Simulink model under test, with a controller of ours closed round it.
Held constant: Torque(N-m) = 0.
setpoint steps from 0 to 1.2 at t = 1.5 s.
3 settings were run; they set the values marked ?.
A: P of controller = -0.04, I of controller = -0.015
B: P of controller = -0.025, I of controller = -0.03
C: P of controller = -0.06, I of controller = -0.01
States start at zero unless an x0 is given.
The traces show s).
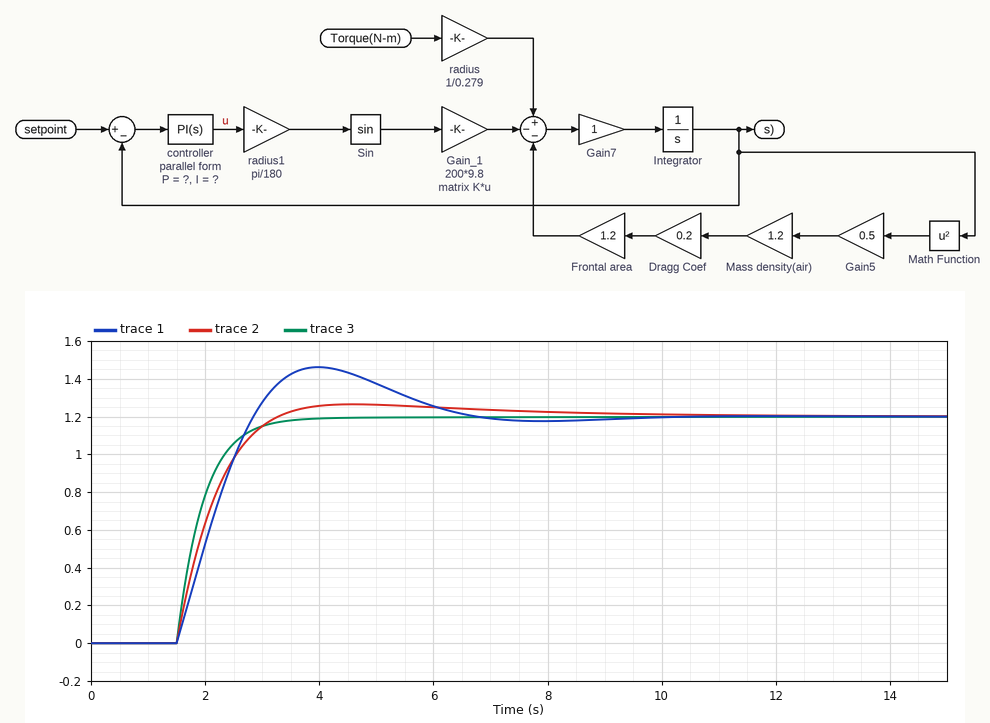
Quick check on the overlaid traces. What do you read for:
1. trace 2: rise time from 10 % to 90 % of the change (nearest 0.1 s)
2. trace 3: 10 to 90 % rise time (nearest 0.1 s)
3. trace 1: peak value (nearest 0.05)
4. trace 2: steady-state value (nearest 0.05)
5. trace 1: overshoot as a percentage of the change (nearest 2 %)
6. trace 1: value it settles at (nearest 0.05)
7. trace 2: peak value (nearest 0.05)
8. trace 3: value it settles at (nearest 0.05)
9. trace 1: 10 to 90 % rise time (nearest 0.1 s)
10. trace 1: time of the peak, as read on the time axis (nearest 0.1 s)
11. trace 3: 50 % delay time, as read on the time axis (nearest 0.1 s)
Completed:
1.2 s
1.0 s
1.45
1.20
22 %
1.20
1.25
1.20
1.0 s
4.0 s
1.8 s
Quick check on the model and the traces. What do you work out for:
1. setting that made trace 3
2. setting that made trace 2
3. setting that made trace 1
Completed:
C
A
B
